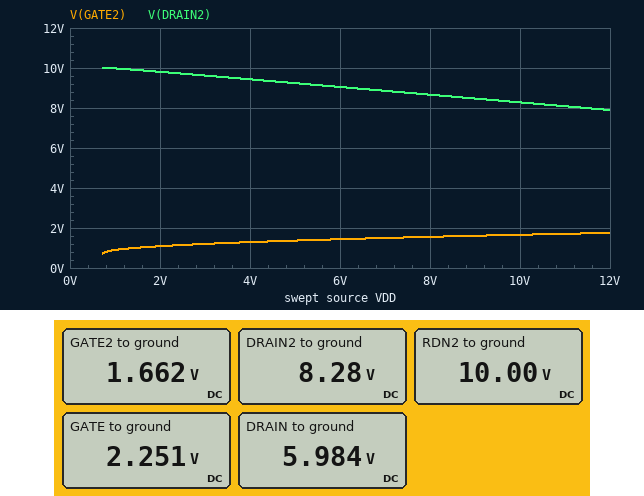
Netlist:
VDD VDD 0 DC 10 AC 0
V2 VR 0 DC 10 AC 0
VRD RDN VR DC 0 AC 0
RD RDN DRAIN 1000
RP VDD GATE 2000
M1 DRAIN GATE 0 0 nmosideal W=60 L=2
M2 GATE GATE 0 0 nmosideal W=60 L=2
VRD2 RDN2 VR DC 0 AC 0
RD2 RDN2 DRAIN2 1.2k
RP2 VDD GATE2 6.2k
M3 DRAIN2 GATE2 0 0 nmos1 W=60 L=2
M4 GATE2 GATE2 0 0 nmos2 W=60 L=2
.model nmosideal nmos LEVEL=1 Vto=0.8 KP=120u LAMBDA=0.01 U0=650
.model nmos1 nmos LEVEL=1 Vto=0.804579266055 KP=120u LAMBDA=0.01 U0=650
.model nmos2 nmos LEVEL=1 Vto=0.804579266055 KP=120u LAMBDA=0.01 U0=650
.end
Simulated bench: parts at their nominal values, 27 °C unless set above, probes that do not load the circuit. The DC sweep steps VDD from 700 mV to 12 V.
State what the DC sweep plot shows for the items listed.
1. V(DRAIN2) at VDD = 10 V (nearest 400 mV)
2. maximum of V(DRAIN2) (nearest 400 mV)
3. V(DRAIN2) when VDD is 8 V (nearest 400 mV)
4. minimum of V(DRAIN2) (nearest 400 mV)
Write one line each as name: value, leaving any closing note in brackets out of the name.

V(DRAIN2) at VDD = 10 V: 8.4 V
maximum of V(DRAIN2): 10.0 V
V(DRAIN2) when VDD is 8 V: 8.8 V
minimum of V(DRAIN2): 8.0 V
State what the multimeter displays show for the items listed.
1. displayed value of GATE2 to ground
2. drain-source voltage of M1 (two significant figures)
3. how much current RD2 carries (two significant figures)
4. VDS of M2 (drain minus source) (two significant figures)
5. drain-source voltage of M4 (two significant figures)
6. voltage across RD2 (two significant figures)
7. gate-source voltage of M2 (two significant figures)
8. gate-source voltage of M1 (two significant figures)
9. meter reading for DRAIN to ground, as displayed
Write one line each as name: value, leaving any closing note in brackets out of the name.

displayed value of GATE2 to ground: 1.662 V
drain-source voltage of M1: 6.0 V
how much current RD2 carries: 1.4 mA
VDS of M2 (drain minus source): 2.3 V
drain-source voltage of M4: 1.7 V
voltage across RD2: 1.7 V
gate-source voltage of M2: 2.3 V
gate-source voltage of M1: 2.3 V
meter reading for DRAIN to ground, as displayed: 5.984 V
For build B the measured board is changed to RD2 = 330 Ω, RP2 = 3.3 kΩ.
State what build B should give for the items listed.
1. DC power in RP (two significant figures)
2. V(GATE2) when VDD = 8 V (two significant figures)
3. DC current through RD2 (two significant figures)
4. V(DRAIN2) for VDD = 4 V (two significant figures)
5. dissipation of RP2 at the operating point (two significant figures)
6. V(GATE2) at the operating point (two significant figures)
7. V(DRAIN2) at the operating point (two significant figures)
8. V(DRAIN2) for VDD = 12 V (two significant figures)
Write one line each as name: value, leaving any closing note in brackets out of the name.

DC power in RP: 30 mW
V(GATE2) when VDD = 8 V: 1.8 V
DC current through RD2: 2.6 mA
V(DRAIN2) for VDD = 4 V: 9.7 V
dissipation of RP2 at the operating point: 20 mW
V(GATE2) at the operating point: 2.0 V
V(DRAIN2) at the operating point: 9.1 V
V(DRAIN2) for VDD = 12 V: 8.9 V
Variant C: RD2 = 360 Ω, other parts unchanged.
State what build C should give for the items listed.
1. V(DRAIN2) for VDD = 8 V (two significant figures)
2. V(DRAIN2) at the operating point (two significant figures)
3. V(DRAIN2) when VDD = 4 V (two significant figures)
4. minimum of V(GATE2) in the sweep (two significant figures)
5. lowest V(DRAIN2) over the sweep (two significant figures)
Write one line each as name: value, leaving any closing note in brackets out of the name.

V(DRAIN2) for VDD = 8 V: 9.6 V
V(DRAIN2) at the operating point: 9.5 V
V(DRAIN2) when VDD = 4 V: 9.8 V
minimum of V(GATE2) in the sweep: 700 mV
lowest V(DRAIN2) over the sweep: 9.4 V
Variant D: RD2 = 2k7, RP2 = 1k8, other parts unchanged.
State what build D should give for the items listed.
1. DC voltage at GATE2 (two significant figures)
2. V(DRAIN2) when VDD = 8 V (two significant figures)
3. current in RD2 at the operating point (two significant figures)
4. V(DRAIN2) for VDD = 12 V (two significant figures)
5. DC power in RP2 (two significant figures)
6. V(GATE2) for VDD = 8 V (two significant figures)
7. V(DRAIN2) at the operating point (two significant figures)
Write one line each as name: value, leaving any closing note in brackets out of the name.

DC voltage at GATE2: 2.3 V
V(DRAIN2) when VDD = 8 V: 1.3 V
current in RD2 at the operating point: 3.4 mA
V(DRAIN2) for VDD = 12 V: 710 mV
DC power in RP2: 33 mW
V(GATE2) for VDD = 8 V: 2.1 V
V(DRAIN2) at the operating point: 850 mV
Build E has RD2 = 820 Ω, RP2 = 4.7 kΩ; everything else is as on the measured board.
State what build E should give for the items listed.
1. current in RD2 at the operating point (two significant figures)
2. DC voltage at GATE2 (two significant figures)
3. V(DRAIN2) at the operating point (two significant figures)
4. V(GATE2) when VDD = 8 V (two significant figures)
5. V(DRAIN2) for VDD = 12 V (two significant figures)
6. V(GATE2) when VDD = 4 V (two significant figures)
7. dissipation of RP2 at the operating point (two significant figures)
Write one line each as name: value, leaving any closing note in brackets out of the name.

current in RD2 at the operating point: 1.9 mA
DC voltage at GATE2: 1.8 V
V(DRAIN2) at the operating point: 8.5 V
V(GATE2) when VDD = 8 V: 1.7 V
V(DRAIN2) for VDD = 12 V: 8.1 V
V(GATE2) when VDD = 4 V: 1.4 V
dissipation of RP2 at the operating point: 14 mW
